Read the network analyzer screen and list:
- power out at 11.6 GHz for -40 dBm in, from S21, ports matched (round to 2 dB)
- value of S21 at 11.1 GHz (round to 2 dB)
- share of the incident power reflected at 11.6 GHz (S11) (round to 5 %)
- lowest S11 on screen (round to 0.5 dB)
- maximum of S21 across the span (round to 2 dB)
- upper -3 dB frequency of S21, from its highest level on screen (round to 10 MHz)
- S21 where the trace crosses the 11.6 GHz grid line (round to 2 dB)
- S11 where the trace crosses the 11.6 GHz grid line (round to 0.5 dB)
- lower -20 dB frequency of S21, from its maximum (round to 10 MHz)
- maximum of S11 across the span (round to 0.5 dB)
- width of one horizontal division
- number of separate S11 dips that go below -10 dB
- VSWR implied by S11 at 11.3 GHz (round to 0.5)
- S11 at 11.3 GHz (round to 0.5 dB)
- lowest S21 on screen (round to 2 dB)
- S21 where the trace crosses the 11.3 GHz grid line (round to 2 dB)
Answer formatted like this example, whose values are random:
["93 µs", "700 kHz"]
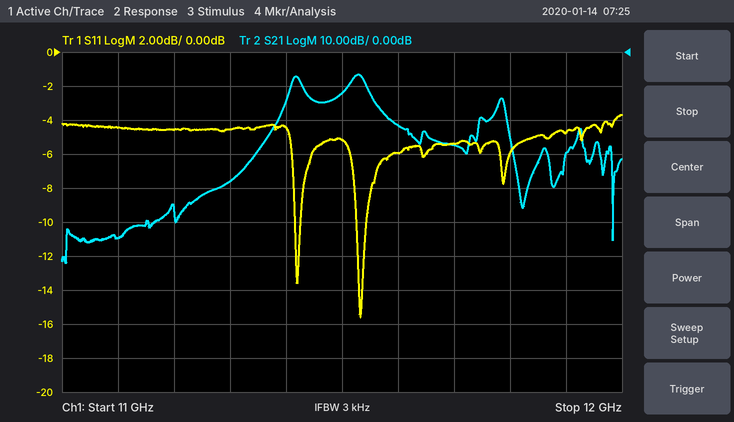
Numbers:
["-62 dBm", "-54 dB", "25 %", "-15.5 dB", "-6 dB", "11.54 GHz", "-22 dB", "-6.0 dB", "11.36 GHz", "-3.5 dB", "100 MHz", "2", "4.0", "-4.5 dB", "-62 dB", "-38 dB"]
